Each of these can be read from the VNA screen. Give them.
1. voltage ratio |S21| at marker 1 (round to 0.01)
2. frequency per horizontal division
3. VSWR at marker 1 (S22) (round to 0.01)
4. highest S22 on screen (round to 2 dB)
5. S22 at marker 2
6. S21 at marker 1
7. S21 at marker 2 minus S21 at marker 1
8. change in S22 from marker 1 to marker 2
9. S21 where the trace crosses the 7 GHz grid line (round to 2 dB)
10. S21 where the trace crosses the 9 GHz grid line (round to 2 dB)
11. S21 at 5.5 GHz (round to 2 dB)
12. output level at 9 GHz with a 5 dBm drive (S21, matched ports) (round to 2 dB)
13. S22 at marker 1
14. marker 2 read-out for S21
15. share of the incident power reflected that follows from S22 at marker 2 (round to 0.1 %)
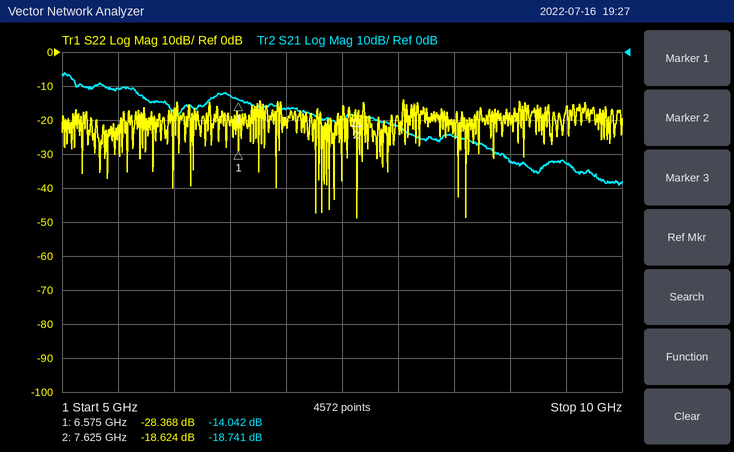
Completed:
0.20
500 MHz
1.08
-14 dB
-18.624 dB
-14.042 dB
-4.699 dB
9.744 dB
-16 dB
-32 dB
-10 dB
-28 dBm
-28.368 dB
-18.741 dB
1.4 %
